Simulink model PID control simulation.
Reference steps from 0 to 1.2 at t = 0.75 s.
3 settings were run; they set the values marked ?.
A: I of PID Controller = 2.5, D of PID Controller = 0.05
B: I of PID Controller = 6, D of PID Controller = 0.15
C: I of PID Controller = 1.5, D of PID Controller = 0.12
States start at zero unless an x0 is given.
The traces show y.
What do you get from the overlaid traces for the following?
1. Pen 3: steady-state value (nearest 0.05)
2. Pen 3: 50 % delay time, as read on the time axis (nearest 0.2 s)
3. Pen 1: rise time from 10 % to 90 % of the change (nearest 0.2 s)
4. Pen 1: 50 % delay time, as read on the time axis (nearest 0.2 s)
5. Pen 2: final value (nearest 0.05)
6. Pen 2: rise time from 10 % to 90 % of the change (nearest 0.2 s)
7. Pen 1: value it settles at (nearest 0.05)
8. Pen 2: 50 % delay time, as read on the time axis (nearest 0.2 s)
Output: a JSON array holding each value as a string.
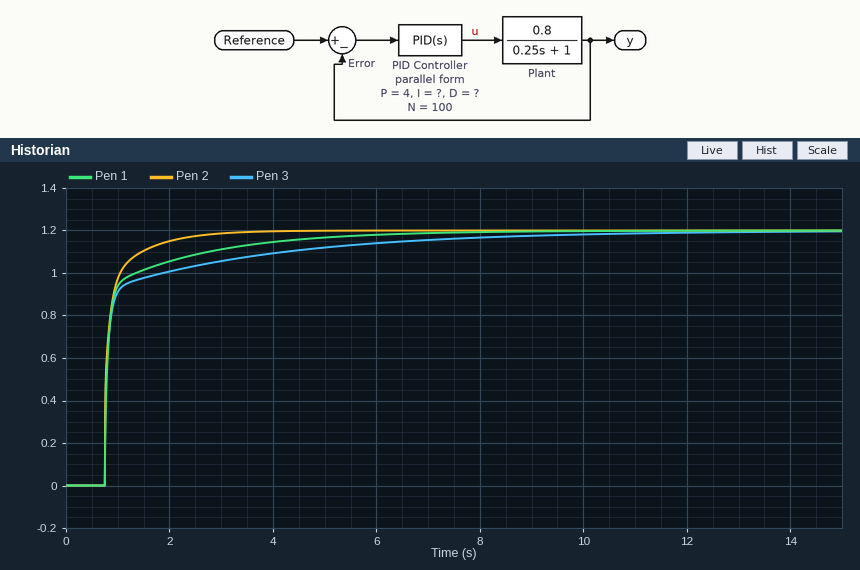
["1.20", "0.8 s", "1.6 s", "0.8 s", "1.20", "0.6 s", "1.20", "0.8 s"]
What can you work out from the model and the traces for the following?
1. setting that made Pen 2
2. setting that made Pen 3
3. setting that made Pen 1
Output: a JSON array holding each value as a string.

["B", "C", "A"]
